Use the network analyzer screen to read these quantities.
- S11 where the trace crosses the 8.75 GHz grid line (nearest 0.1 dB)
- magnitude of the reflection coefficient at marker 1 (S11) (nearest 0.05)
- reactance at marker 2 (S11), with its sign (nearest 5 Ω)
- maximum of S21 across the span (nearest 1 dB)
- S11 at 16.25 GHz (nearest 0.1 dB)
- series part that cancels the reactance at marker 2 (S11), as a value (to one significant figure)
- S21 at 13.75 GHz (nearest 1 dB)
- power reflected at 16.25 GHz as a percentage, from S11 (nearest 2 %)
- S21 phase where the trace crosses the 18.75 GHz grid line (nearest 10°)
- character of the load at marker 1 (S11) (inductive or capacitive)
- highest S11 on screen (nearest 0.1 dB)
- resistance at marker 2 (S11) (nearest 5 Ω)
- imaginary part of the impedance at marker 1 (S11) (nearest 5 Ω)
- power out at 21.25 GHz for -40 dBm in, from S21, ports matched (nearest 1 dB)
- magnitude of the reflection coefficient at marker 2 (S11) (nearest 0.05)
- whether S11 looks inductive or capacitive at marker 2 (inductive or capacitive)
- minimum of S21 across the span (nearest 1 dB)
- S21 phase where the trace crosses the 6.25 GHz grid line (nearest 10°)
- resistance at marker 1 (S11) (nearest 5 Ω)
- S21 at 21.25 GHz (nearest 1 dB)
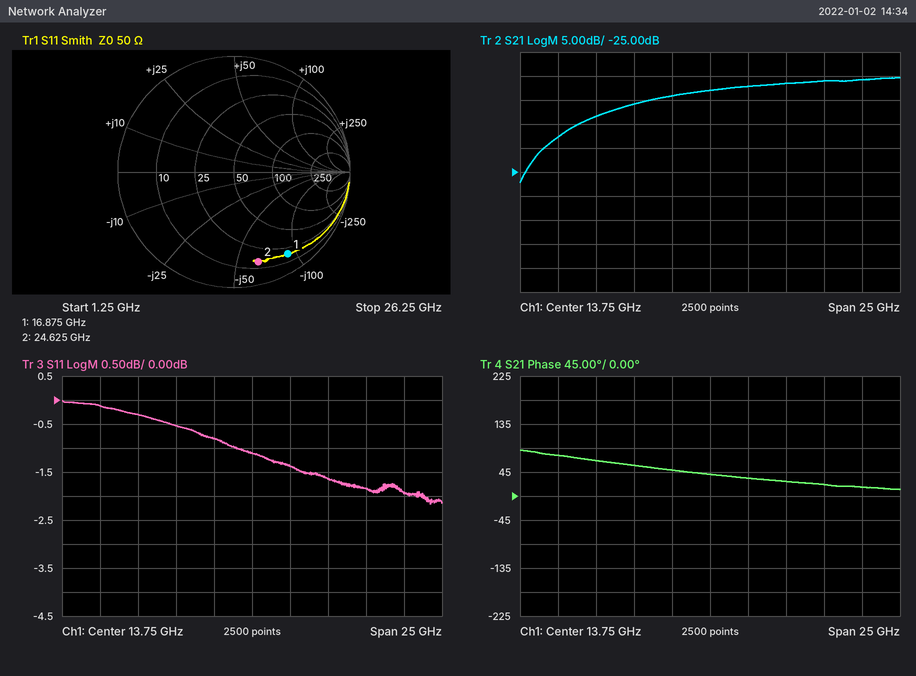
-0.5 dB
0.85
-65 Ω
-5 dB
-1.4 dB
400 pH
-8 dB
72 %
30°
capacitive
0.0 dB
15 Ω
-90 Ω
-46 dBm
0.80
capacitive
-27 dB
70°
20 Ω
-6 dB
